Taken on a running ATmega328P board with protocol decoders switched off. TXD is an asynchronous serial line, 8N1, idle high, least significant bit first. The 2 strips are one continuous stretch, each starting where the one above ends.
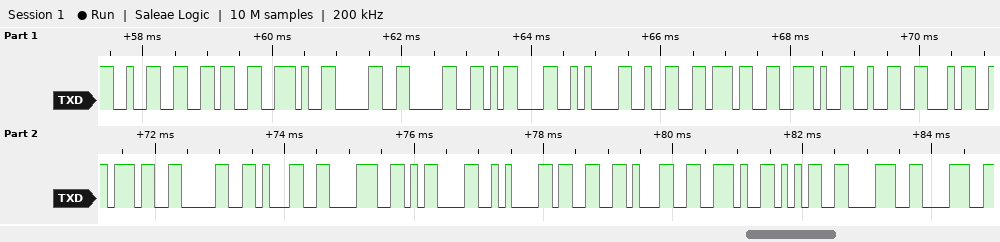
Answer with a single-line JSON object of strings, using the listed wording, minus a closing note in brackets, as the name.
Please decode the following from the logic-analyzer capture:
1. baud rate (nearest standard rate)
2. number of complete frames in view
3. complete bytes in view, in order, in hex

{"baud rate": "9600 baud", "number of complete frames in view": "24", "complete bytes in view, in order, in hex": "32 36 2E 30 30 0D 0A 32 37 2E 32 34 37 30 31 38 0D 0A 33 31 2E 35 38 38"}
